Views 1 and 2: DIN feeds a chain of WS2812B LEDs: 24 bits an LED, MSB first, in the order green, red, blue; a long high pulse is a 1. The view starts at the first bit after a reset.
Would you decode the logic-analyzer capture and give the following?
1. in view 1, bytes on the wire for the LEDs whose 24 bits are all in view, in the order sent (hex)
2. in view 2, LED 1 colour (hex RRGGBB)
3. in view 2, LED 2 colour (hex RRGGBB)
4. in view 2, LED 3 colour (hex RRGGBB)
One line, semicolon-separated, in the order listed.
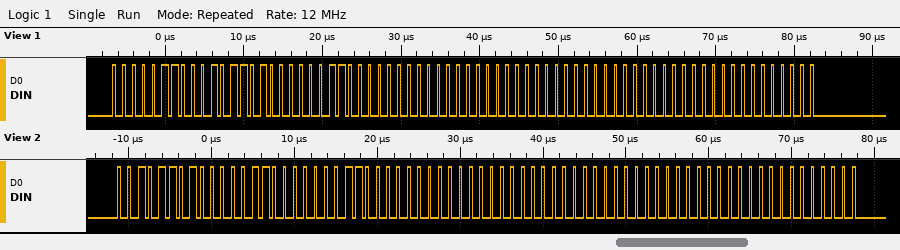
06 2D 03 00 00 00 00 00 00; #062D03; #000000; #000000
